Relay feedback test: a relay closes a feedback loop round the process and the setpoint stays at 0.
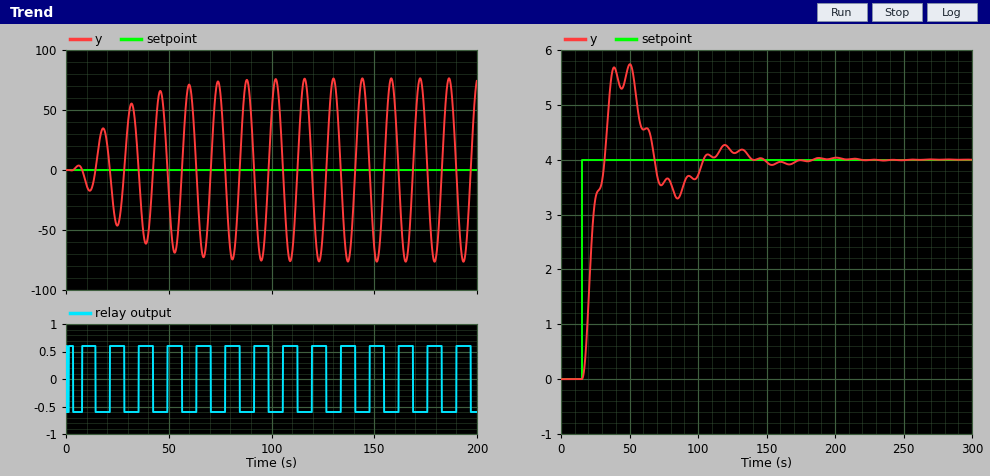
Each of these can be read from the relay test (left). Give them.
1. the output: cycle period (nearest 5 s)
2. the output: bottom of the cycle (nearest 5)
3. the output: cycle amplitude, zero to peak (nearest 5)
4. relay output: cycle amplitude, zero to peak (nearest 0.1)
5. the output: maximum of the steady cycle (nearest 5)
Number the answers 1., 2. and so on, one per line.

1. 15 s
2. -75
3. 75
4. 0.6
5. 75
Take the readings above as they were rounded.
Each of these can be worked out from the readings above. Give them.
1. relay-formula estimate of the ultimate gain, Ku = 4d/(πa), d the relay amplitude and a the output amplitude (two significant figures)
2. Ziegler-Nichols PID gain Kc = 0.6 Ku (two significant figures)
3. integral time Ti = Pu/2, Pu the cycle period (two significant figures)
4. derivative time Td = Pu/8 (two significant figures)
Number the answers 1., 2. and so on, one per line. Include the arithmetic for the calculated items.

1. 4 × 0.6 / (π × 75) = 0.010
2. 0.6 × 0.01 = 0.0060
3. 15 / 2 = 7.5 s
4. 15 / 8 = 1.9 s
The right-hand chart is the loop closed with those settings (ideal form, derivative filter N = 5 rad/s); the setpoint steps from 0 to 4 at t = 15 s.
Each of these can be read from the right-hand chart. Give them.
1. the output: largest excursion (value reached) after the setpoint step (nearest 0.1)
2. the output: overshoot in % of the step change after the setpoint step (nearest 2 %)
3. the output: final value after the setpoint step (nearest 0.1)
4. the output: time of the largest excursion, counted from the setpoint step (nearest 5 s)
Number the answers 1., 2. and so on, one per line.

1. 5.7
2. 44 %
3. 4.0
4. 35 s
